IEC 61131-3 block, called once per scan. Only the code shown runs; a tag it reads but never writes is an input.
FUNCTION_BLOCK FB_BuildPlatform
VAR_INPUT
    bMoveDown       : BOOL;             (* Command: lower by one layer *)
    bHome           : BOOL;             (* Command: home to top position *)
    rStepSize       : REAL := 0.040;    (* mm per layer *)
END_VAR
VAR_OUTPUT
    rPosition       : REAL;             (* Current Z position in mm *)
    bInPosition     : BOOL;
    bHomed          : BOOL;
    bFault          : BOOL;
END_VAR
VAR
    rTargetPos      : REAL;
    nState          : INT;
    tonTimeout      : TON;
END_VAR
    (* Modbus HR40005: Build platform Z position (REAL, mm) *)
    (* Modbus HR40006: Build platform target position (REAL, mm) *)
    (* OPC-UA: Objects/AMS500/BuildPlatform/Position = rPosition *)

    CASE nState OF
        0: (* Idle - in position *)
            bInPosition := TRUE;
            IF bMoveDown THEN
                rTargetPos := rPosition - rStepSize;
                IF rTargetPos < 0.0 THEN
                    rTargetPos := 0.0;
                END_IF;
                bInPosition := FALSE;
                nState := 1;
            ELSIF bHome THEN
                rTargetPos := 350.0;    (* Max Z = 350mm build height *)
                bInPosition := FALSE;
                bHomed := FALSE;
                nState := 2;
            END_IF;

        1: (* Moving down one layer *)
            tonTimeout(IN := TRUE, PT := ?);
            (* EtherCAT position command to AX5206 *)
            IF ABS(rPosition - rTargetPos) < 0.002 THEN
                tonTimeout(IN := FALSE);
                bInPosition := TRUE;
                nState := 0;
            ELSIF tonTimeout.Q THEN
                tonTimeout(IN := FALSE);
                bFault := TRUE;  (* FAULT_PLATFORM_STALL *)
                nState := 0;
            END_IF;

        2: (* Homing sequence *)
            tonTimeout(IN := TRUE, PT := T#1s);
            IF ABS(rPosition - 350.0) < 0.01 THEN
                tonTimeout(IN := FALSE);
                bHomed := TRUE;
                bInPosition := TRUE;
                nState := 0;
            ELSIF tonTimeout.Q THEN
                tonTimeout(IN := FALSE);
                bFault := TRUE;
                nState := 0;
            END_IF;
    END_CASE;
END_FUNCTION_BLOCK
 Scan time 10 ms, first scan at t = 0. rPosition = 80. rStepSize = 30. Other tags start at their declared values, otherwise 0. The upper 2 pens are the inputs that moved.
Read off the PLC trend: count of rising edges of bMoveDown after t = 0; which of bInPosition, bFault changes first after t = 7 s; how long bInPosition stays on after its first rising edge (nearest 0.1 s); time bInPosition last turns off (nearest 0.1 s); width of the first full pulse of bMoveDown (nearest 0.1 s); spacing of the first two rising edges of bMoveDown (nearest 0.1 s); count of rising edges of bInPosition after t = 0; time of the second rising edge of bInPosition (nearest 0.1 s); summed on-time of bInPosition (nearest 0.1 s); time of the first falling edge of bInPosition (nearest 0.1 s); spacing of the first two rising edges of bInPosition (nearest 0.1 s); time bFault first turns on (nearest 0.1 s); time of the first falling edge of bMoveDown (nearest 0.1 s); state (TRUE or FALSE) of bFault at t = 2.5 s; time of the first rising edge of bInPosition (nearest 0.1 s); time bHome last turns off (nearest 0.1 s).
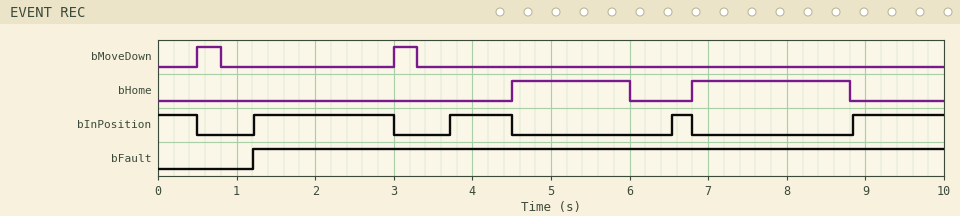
2
bInPosition
1.8 s
6.8 s
0.3 s
2.5 s
4
3.7 s
4.5 s
0.5 s
2.5 s
1.2 s
0.8 s
TRUE
1.2 s
8.8 s
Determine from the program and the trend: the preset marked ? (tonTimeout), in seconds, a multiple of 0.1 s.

0.7 s
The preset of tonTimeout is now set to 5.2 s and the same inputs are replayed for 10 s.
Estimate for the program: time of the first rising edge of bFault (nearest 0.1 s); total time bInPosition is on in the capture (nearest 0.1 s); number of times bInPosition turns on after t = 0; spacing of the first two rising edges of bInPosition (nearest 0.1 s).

5.7 s
1.7 s
2
2.1 s
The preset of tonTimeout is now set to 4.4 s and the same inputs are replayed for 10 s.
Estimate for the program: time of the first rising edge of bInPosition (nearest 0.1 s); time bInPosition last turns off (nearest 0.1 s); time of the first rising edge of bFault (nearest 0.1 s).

9.0 s
0.5 s
4.9 s
